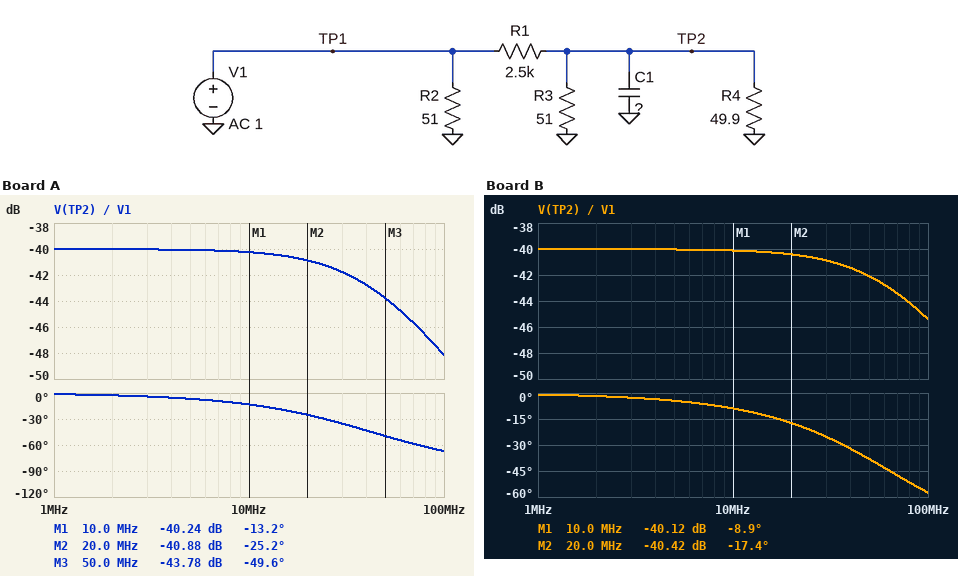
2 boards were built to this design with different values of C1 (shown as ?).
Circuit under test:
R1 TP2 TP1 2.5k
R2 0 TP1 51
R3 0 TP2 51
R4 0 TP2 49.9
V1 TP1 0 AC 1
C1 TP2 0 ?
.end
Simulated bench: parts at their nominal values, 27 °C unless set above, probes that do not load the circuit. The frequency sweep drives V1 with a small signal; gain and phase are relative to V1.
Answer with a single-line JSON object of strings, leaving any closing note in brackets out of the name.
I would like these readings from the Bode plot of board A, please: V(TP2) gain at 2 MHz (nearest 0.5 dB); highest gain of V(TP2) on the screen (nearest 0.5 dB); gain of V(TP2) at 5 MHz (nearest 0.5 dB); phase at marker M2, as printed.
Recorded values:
{"V(TP2) gain at 2 MHz": "-40.0 dB", "highest gain of V(TP2) on the screen": "-40.0 dB", "gain of V(TP2) at 5 MHz": "-40.0 dB", "phase at marker M2, as printed": "-25.2 deg"}
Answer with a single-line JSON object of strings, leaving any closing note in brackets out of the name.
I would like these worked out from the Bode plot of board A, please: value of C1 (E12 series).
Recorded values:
{"value of C1": "150 pF"}
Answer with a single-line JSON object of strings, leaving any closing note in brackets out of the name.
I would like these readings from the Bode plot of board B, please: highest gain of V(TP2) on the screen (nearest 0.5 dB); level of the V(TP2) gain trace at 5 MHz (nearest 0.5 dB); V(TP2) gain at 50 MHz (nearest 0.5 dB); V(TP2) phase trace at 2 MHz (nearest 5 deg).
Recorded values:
{"highest gain of V(TP2) on the screen": "-40.0 dB", "level of the V(TP2) gain trace at 5 MHz": "-40.0 dB", "V(TP2) gain at 50 MHz": "-42.0 dB", "V(TP2) phase trace at 2 MHz": "0 deg"}
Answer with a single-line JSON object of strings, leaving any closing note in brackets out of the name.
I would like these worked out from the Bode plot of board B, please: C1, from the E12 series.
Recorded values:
{"C1, from the E12 series": "100 pF"}
